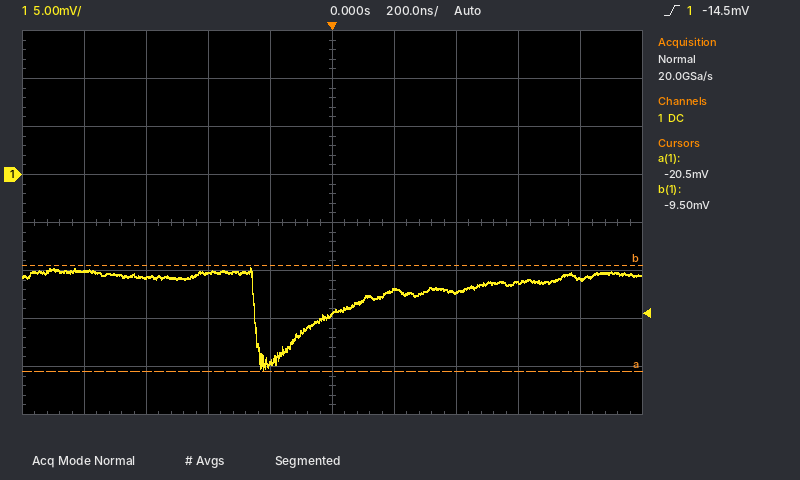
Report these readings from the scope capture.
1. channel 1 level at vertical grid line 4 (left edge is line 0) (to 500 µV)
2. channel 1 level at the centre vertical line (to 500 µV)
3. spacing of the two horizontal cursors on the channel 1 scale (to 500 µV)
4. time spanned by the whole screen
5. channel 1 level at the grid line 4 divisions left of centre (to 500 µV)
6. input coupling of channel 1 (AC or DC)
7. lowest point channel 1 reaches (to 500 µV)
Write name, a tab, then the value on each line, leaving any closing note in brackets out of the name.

channel 1 level at vertical grid line 4 (left edge is line 0)	-19.5 mV
channel 1 level at the centre vertical line	-14.5 mV
spacing of the two horizontal cursors on the channel 1 scale	11.0 mV
time spanned by the whole screen	2 µs
channel 1 level at the grid line 4 divisions left of centre	-10.0 mV
input coupling of channel 1	DC
lowest point channel 1 reaches	-20.5 mV
